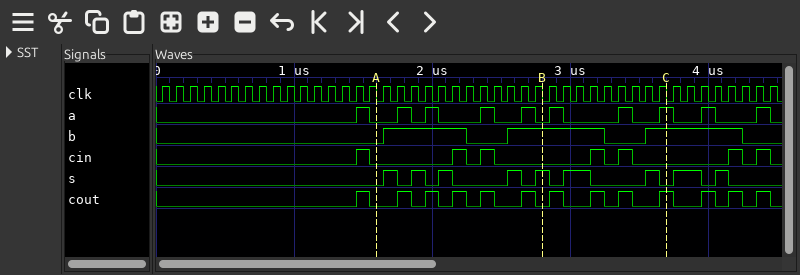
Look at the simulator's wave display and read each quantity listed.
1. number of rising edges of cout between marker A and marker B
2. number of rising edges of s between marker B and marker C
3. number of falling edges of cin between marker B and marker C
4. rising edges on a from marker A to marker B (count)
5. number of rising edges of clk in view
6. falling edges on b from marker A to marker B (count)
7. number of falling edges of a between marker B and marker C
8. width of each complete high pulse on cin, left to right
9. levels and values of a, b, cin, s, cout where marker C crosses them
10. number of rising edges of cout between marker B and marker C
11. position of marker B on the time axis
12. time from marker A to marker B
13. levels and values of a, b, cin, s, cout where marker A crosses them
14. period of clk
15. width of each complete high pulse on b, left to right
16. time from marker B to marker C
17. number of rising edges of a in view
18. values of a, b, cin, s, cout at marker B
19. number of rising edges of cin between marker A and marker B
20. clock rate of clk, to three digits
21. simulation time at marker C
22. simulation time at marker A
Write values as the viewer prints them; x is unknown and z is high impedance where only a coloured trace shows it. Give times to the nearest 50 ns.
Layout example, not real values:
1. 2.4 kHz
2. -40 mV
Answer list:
1. 5
2. 2
3. 2
4. 4
5. 45
6. 1
7. 2
8. 100 ns, 100 ns, 100 ns, 100 ns, 100 ns, 100 ns, 100 ns
9. a=1, b=1, cin=0, s=0, cout=1
10. 4
11. 2800 ns
12. 1200 ns
13. a=0, b=0, cin=0, s=0, cout=0
14. 100 ns
15. 600 ns, 700 ns, 700 ns
16. 900 ns
17. 10
18. a=0, b=1, cin=0, s=1, cout=0
19. 2
20. 10.0 MHz
21. 3700 ns
22. 1600 ns
